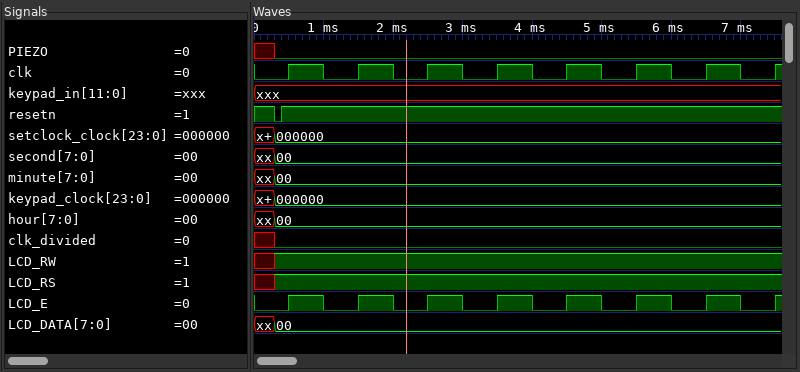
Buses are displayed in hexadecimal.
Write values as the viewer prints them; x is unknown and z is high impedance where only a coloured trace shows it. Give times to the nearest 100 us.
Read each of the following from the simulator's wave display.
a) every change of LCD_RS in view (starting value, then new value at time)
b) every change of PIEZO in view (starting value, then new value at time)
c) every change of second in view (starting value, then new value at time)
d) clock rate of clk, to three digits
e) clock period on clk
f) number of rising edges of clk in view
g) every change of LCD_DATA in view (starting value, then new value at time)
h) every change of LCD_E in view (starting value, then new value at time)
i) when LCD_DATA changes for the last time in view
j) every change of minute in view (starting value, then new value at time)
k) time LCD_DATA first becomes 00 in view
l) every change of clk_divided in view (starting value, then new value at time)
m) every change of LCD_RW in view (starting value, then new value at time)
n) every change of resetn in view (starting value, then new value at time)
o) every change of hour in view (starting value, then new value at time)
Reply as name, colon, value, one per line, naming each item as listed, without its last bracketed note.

every change of LCD_RS in view: x, 1 at 300 us
every change of PIEZO in view: x, 0 at 300 us
every change of second in view: xx, 00 at 300 us
clock rate of clk, to three digits: 1.00 kHz
clock period on clk: 1000 us
number of rising edges of clk in view: 8
every change of LCD_DATA in view: xx, 00 at 300 us
every change of LCD_E in view: 0, 1 at 500 us, 0 at 1000 us, 1 at 1500 us, 0 at 2000 us, 1 at 2500 us, 0 at 3000 us, 1 at 3500 us, 0 at 4000 us, 1 at 4500 us, 0 at 5000 us, 1 at 5500 us, 0 at 6000 us, 1 at 6500 us, 0 at 7000 us, 1 at 7500 us
when LCD_DATA changes for the last time in view: 300 us
every change of minute in view: xx, 00 at 300 us
time LCD_DATA first becomes 00 in view: 300 us
every change of clk_divided in view: x, 0 at 300 us
every change of LCD_RW in view: x, 1 at 300 us
every change of resetn in view: 1, 0 at 300 us, 1 at 400 us
every change of hour in view: xx, 00 at 300 us
